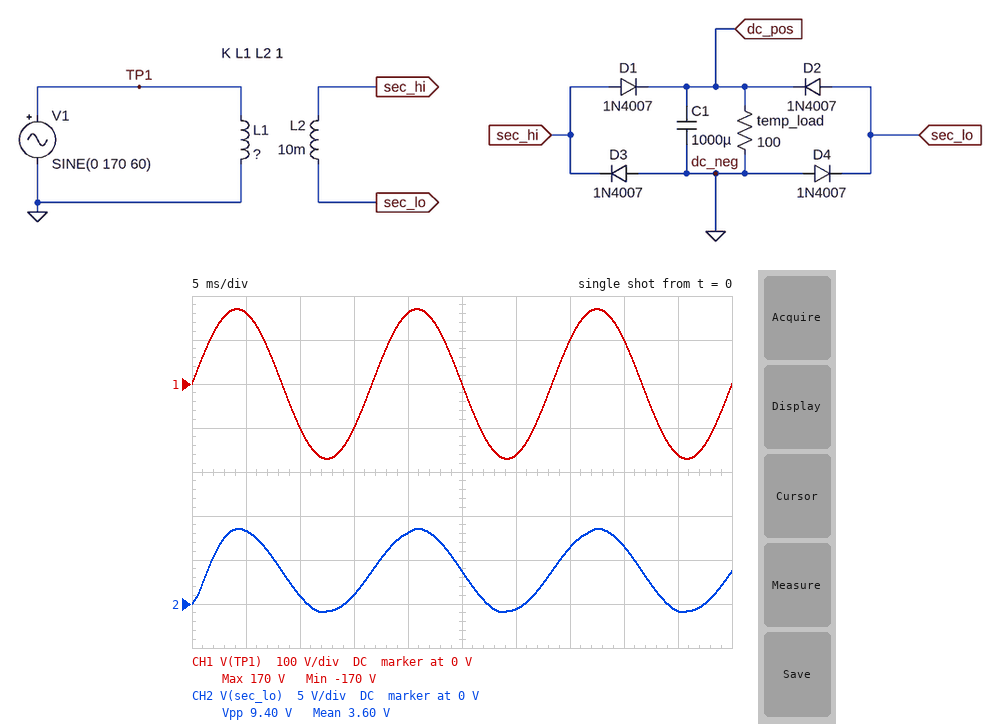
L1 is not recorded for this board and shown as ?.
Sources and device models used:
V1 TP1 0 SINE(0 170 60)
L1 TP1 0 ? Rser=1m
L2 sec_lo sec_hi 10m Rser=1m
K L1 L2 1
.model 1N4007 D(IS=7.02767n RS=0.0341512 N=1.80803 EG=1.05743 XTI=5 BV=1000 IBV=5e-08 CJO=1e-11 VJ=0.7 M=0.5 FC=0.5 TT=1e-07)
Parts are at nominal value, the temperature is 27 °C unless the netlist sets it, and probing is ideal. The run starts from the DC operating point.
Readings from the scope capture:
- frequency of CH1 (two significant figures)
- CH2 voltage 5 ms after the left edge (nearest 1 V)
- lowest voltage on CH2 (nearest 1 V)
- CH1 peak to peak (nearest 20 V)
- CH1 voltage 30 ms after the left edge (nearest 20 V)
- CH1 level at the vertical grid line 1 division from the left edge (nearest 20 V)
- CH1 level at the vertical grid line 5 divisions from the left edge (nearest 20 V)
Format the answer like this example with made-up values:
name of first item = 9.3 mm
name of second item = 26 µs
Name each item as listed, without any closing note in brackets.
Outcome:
frequency of CH1 = 60 Hz
CH2 voltage 5 ms after the left edge = 8 V
lowest voltage on CH2 = -1 V
CH1 peak to peak = 340 V
CH1 voltage 30 ms after the left edge = -160 V
CH1 level at the vertical grid line 1 division from the left edge = 160 V
CH1 level at the vertical grid line 5 divisions from the left edge = 0 V
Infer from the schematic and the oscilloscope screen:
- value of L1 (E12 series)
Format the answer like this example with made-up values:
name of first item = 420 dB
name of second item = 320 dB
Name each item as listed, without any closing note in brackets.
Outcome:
value of L1 = 3.3 H
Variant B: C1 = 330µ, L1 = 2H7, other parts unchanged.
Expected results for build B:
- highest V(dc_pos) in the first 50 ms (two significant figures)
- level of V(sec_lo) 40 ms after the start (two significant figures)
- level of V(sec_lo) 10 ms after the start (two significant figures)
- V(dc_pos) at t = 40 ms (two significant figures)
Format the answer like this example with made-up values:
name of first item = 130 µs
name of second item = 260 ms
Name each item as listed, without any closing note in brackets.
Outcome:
highest V(dc_pos) in the first 50 ms = 8.8 V
level of V(sec_lo) 40 ms after the start = 7.2 V
level of V(sec_lo) 10 ms after the start = 680 mV
V(dc_pos) at t = 40 ms = 8.2 V
